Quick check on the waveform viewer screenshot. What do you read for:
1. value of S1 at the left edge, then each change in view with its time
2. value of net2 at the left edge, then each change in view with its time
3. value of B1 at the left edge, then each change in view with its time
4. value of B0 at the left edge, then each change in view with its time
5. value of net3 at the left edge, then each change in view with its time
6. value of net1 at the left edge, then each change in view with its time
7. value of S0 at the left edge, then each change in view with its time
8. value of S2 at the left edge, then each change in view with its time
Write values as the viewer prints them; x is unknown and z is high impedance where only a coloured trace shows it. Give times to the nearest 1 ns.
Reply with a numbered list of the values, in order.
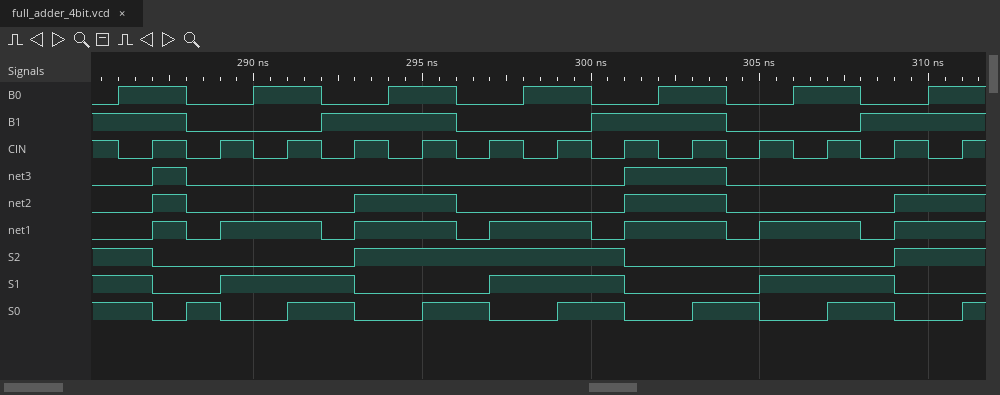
1. 1, 0 at 287 ns, 1 at 289 ns, 0 at 293 ns, 1 at 297 ns, 0 at 301 ns, 1 at 305 ns, 0 at 309 ns
2. 0, 1 at 287 ns, 0 at 288 ns, 1 at 293 ns, 0 at 296 ns, 1 at 301 ns, 0 at 304 ns, 1 at 309 ns
3. 1, 0 at 288 ns, 1 at 292 ns, 0 at 296 ns, 1 at 300 ns, 0 at 304 ns, 1 at 308 ns
4. 0, 1 at 286 ns, 0 at 288 ns, 1 at 290 ns, 0 at 292 ns, 1 at 294 ns, 0 at 296 ns, 1 at 298 ns, 0 at 300 ns, 1 at 302 ns, 0 at 304 ns, 1 at 306 ns, 0 at 308 ns, 1 at 310 ns
5. 0, 1 at 287 ns, 0 at 288 ns, 1 at 301 ns, 0 at 304 ns
6. 0, 1 at 287 ns, 0 at 288 ns, 1 at 289 ns, 0 at 292 ns, 1 at 293 ns, 0 at 296 ns, 1 at 297 ns, 0 at 300 ns, 1 at 301 ns, 0 at 304 ns, 1 at 305 ns, 0 at 308 ns, 1 at 309 ns
7. 1, 0 at 287 ns, 1 at 288 ns, 0 at 289 ns, 1 at 291 ns, 0 at 293 ns, 1 at 295 ns, 0 at 297 ns, 1 at 299 ns, 0 at 301 ns, 1 at 303 ns, 0 at 305 ns, 1 at 307 ns, 0 at 309 ns, 1 at 311 ns
8. 1, 0 at 287 ns, 1 at 293 ns, 0 at 301 ns, 1 at 309 ns
